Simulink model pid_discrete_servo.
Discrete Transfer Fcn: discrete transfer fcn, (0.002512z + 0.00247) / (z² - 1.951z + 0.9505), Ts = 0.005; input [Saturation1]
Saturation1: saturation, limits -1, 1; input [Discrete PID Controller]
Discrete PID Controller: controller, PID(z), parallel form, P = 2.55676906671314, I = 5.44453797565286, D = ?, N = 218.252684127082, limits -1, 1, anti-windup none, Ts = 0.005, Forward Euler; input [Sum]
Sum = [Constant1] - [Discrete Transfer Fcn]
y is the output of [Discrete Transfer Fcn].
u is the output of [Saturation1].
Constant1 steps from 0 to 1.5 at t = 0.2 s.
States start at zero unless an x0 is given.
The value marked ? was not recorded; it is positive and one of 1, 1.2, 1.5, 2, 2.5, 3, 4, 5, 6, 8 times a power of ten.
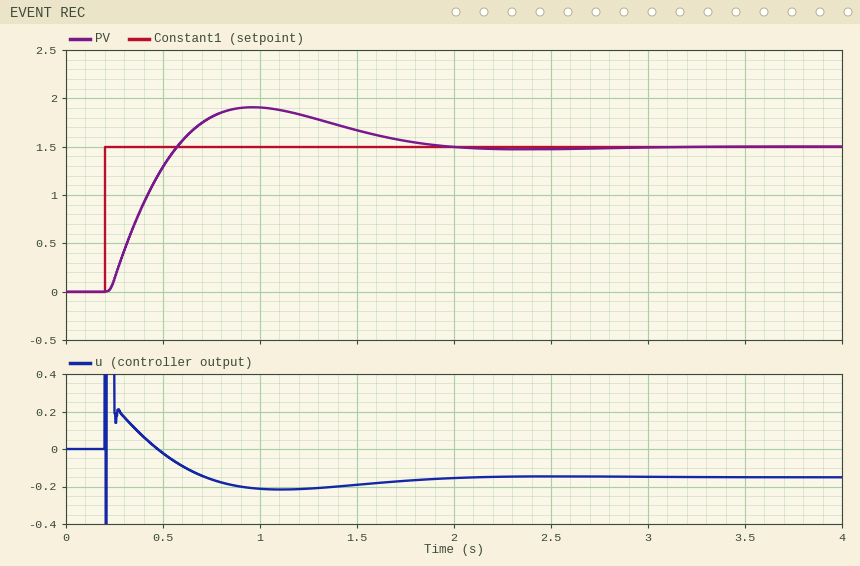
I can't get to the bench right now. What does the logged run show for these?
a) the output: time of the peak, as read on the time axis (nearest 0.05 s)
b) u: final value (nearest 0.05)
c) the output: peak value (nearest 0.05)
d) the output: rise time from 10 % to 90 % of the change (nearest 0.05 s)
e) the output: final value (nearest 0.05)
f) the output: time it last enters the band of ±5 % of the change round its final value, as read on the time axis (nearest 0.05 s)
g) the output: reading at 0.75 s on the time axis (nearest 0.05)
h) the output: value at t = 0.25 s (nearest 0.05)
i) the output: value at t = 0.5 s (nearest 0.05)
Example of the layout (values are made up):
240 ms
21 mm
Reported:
0.95 s
-0.15
1.90
0.25 s
1.50
1.70 s
1.80
0.15
1.30
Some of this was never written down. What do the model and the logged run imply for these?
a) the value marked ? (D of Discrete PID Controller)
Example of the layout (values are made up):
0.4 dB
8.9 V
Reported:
0.6
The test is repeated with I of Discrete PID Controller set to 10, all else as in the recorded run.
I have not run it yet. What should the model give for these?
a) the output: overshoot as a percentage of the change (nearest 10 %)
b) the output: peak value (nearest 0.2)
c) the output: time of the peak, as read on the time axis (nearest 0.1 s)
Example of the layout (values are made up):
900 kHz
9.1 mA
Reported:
40 %
2.0
0.8 s
